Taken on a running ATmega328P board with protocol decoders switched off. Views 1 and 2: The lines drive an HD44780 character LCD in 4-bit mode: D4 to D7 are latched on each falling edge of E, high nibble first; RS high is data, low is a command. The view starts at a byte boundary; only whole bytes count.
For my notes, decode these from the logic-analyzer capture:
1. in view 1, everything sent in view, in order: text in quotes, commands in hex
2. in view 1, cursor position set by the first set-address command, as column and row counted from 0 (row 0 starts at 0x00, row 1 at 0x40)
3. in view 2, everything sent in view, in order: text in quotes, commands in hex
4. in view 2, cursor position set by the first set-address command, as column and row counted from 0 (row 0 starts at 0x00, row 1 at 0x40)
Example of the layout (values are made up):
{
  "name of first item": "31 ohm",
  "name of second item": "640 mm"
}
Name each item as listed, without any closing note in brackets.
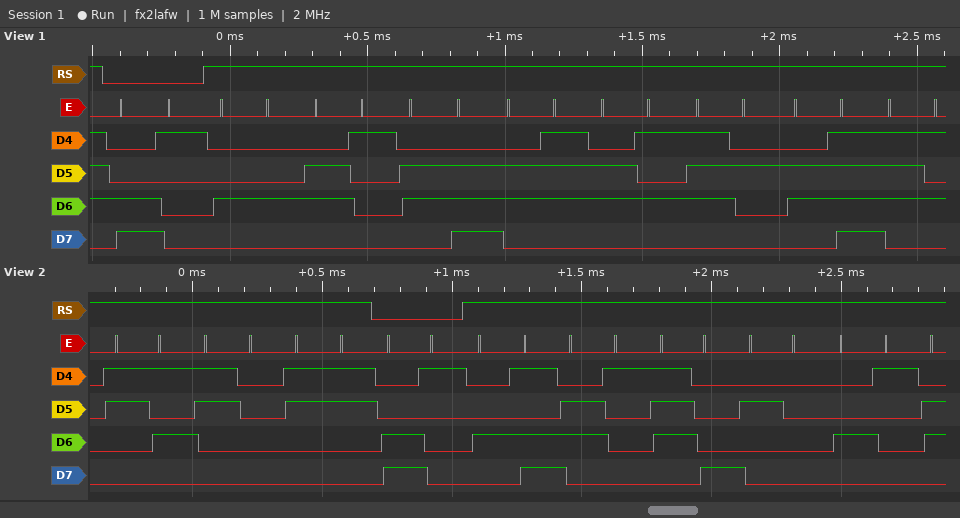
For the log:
{
  "in view 1, everything sent in view, in order: text in quotes, commands in hex": "0xC1 \"Dangerou\"",
  "in view 1, cursor position set by the first set-address command, as column and row counted from 0": "column 1, row 1",
  "in view 2, everything sent in view, in order: text in quotes, commands in hex": "\"503\" 0xC1 \"Max A\"",
  "in view 2, cursor position set by the first set-address command, as column and row counted from 0": "column 1, row 1"
}
